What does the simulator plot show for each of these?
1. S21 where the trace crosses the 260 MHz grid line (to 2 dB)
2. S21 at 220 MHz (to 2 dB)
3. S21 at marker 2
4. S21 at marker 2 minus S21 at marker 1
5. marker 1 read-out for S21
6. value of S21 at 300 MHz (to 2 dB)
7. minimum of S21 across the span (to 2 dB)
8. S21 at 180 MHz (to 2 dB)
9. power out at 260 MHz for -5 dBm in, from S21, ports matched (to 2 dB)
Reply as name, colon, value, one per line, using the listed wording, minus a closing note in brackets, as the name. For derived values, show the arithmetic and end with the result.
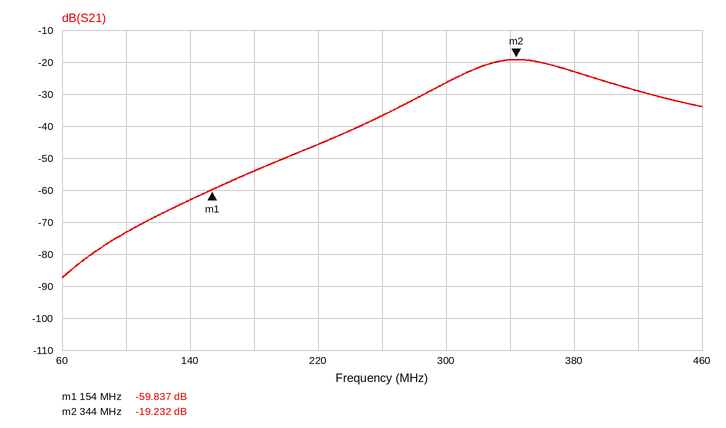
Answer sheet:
S21 where the trace crosses the 260 MHz grid line: -36 dB
S21 at 220 MHz: -46 dB
S21 at marker 2: -19.232 dB
S21 at marker 2 minus S21 at marker 1: -19.232 − (-59.837) = 40.605 dB
marker 1 read-out for S21: -59.837 dB
value of S21 at 300 MHz: -26 dB
minimum of S21 across the span: -88 dB
S21 at 180 MHz: -54 dB
power out at 260 MHz for -5 dBm in, from S21, ports matched: -5 dBm + (-36 dB) = -42 dBm
